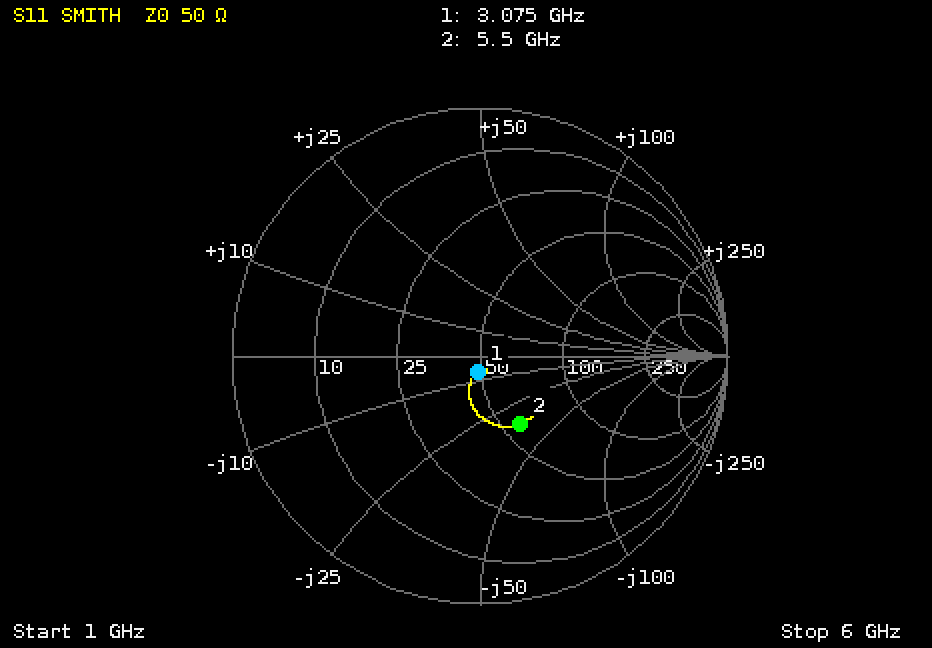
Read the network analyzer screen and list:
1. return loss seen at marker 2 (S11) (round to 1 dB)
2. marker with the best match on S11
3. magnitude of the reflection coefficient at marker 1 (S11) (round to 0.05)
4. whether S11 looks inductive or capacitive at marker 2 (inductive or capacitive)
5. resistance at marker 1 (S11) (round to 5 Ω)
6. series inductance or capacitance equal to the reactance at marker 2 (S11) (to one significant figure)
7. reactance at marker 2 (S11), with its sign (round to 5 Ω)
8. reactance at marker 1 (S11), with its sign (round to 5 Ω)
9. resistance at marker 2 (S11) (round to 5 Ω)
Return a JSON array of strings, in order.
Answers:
["10 dB", "marker 1", "0.05", "capacitive", "50 Ω", "800 fF", "-35 Ω", "-5 Ω", "60 Ω"]
